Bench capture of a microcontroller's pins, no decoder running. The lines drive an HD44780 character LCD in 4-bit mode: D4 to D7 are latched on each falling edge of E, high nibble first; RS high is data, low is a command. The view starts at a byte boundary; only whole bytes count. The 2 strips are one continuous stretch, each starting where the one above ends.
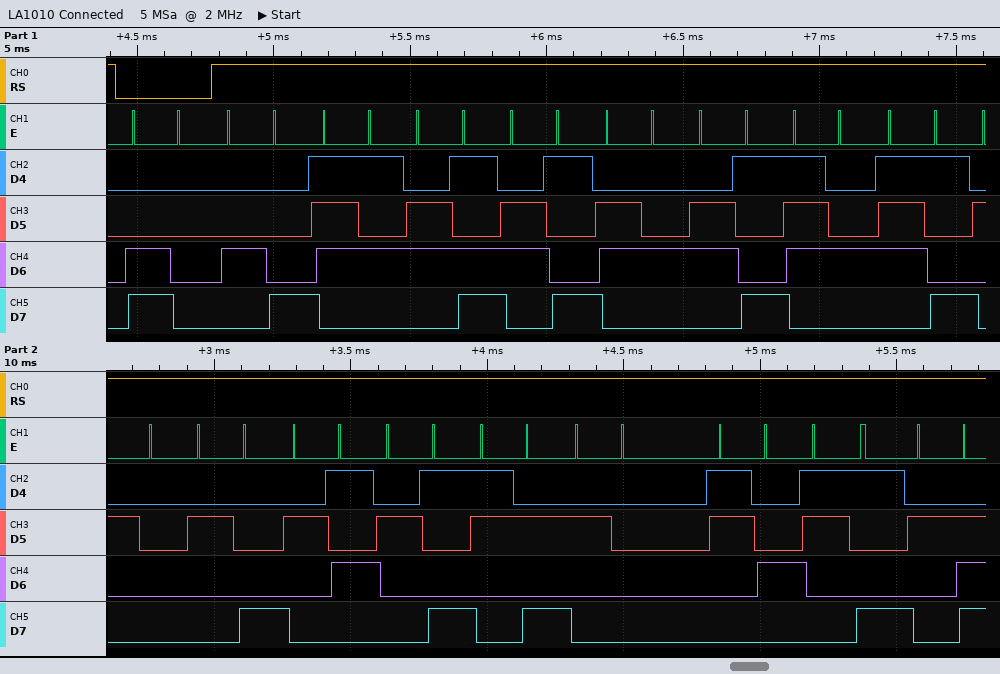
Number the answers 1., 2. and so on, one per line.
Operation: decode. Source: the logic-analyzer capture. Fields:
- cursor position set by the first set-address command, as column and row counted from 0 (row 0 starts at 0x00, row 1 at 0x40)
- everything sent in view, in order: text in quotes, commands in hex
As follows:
1. column 0, row 1
2. 0xC0 "Humidity (%): 49."
